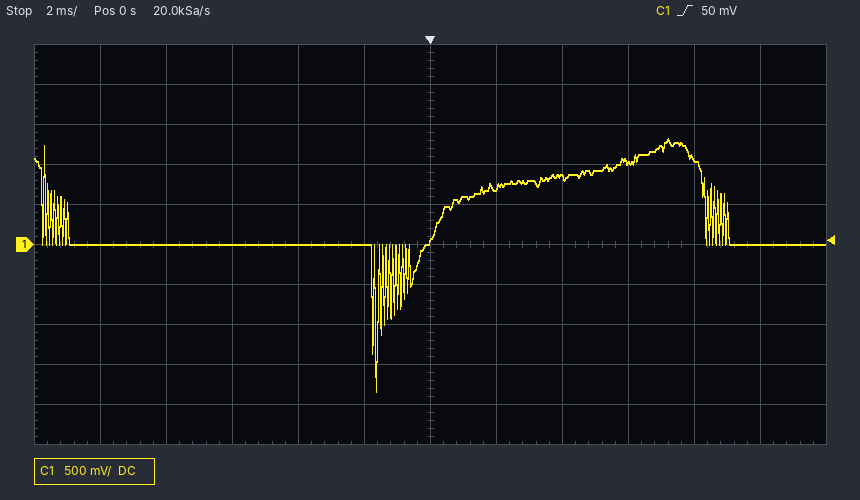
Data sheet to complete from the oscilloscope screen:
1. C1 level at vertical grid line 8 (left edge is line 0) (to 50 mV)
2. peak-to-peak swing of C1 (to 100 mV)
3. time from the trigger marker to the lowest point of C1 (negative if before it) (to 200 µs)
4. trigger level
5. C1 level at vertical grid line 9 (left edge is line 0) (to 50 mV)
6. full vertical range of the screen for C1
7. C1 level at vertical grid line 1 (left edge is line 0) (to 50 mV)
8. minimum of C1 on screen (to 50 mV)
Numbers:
850 mV
3.20 V
-1.6 ms
50 mV
1.05 V
5 V
0 mV
-1.85 V
